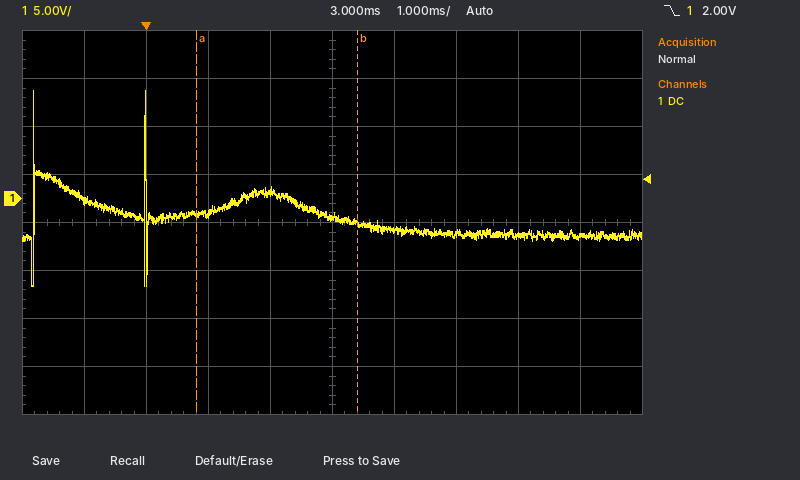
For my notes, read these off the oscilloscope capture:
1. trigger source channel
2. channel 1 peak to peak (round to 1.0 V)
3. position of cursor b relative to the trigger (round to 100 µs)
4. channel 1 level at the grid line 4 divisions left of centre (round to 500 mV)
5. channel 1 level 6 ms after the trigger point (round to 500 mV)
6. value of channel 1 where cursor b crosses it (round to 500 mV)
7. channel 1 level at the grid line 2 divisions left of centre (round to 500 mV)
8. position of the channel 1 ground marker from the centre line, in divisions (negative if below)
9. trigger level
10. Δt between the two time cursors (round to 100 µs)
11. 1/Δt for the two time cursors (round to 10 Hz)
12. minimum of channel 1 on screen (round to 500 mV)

channel 1
20.0 V
+3.4 ms
0.0 V
-4.0 V
-2.5 V
-1.5 V
+0.5 div
2.00 V
2.6 ms
380 Hz
-9.0 V
